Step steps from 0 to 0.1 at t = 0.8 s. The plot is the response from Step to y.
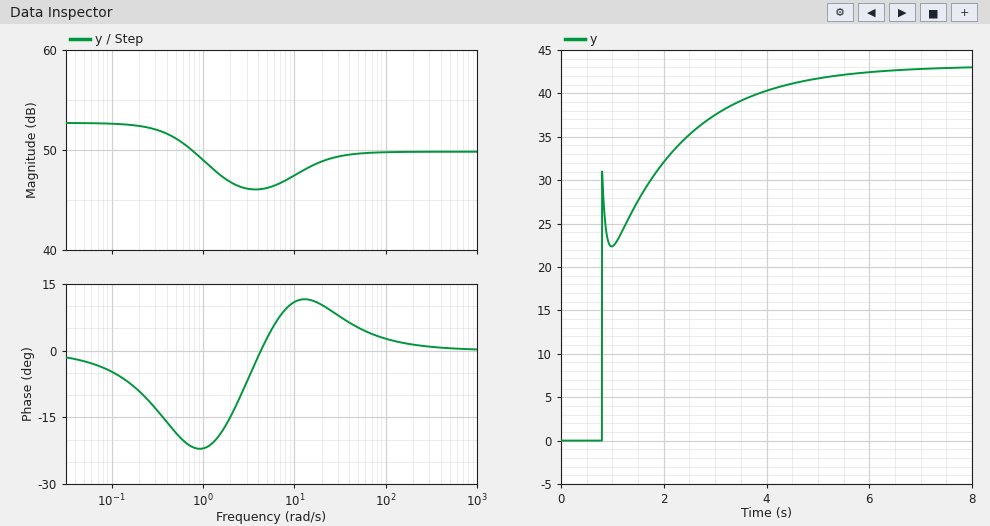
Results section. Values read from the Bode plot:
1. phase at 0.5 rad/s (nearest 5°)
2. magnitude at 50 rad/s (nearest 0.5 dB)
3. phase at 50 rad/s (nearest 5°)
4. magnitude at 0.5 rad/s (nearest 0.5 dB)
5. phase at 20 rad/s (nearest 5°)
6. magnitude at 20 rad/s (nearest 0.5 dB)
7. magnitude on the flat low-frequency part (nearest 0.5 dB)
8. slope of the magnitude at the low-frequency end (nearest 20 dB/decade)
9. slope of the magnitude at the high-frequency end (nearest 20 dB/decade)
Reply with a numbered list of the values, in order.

1. -20°
2. 49.5 dB
3. 5°
4. 51.0 dB
5. 10°
6. 49.0 dB
7. 52.5 dB
8. 0 dB/decade
9. 0 dB/decade
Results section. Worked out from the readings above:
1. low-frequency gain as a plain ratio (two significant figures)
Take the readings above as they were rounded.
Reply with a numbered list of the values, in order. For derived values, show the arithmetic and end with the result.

1. 10^(52.5 / 20) = 420
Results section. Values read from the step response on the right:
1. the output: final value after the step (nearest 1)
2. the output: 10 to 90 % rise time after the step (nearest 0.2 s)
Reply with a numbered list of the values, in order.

1. 43
2. 2.6 s
